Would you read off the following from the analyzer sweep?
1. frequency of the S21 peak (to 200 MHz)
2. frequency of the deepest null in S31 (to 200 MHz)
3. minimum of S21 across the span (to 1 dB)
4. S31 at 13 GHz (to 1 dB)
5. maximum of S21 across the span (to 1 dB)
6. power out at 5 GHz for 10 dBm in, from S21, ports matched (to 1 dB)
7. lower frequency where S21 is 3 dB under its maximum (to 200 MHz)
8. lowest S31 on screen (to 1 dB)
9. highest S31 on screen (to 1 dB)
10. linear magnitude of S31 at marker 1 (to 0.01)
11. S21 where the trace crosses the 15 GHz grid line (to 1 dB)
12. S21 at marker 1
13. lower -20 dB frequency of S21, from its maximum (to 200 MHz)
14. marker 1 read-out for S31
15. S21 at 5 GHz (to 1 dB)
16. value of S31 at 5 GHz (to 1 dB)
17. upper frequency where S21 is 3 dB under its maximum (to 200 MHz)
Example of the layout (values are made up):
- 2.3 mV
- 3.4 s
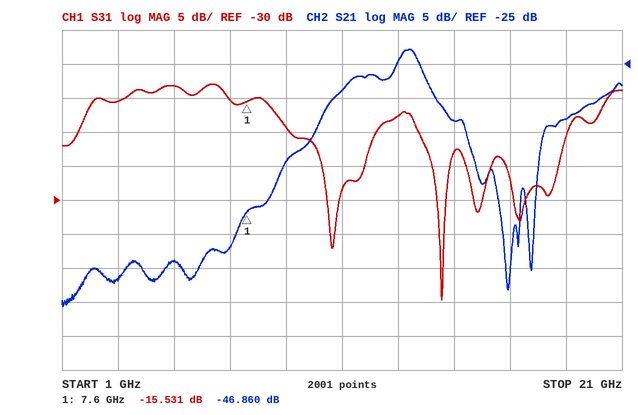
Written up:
- 13.4 GHz
- 14.6 GHz
- -61 dB
- -18 dB
- -23 dB
- -44 dBm
- 12.8 GHz
- -45 dB
- -13 dB
- 0.17
- -33 dB
- -46.860 dB
- 8.6 GHz
- -15.531 dB
- -54 dB
- -13 dB
- 13.8 GHz
